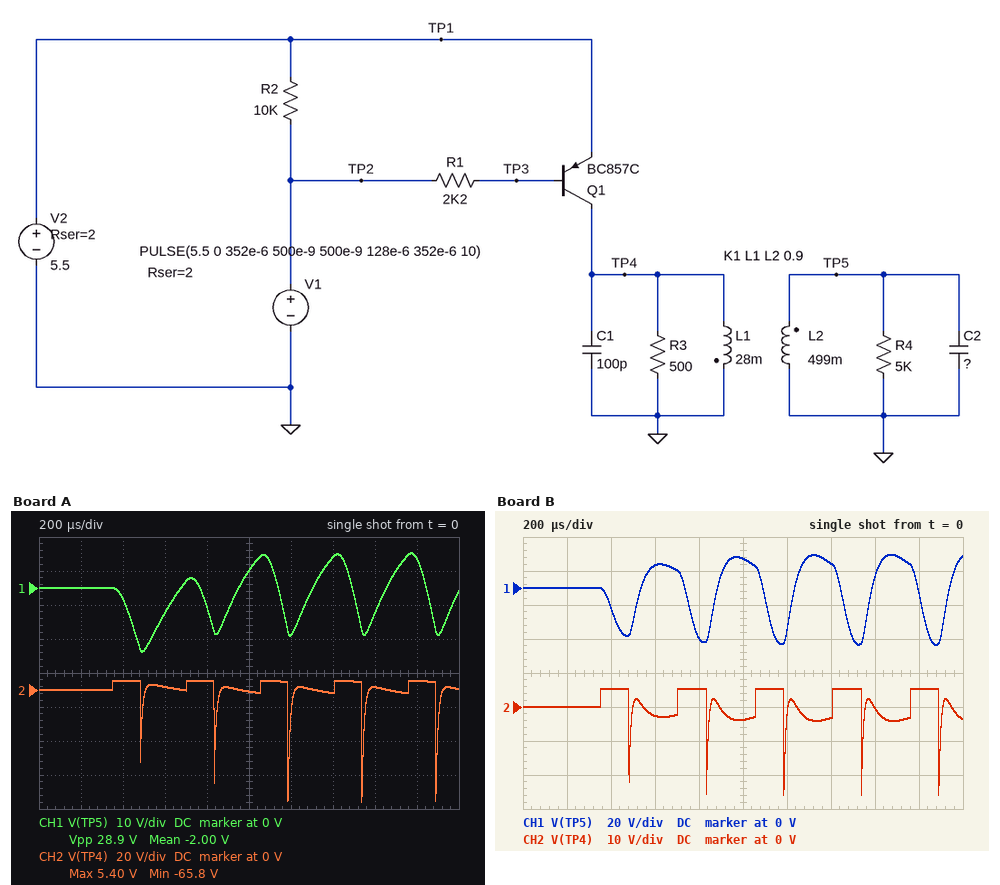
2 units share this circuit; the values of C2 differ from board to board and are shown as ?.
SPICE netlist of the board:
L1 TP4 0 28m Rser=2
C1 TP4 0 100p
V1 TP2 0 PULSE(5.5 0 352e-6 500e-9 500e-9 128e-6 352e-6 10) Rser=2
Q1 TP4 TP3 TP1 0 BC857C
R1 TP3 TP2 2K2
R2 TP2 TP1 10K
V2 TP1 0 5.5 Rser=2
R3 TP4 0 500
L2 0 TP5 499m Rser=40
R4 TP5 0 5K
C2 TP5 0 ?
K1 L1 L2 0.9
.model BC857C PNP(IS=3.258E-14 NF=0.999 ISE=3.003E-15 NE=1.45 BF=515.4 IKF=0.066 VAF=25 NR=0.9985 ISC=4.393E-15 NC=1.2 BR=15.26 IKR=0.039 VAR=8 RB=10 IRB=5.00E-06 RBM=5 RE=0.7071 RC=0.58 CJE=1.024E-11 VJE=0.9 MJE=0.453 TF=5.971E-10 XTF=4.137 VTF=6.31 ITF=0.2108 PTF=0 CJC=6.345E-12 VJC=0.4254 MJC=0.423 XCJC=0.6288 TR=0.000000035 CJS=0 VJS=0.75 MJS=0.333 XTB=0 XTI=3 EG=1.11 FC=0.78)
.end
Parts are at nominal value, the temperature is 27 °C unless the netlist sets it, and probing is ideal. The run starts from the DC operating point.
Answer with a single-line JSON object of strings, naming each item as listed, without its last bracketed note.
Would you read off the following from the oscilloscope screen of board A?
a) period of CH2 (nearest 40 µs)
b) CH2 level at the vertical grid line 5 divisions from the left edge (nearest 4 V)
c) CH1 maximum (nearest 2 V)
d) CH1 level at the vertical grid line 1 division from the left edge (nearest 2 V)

{"period of CH2": "360 µs", "CH2 level at the vertical grid line 5 divisions from the left edge": "0 V", "CH1 maximum": "10 V", "CH1 level at the vertical grid line 1 division from the left edge": "0 V"}
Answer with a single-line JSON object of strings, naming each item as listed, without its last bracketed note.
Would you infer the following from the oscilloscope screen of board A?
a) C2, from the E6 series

{"C2, from the E6 series": "68 nF"}
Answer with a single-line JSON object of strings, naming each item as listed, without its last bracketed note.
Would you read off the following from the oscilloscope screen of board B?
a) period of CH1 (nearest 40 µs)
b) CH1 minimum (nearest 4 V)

{"period of CH1": "360 µs", "CH1 minimum": "-32 V"}
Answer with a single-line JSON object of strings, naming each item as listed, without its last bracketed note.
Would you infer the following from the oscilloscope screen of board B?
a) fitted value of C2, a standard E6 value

{"fitted value of C2, a standard E6 value": "15 nF"}
